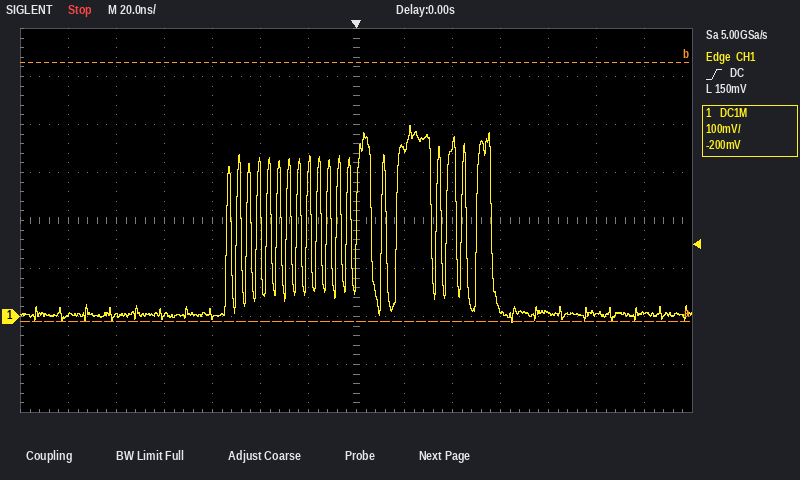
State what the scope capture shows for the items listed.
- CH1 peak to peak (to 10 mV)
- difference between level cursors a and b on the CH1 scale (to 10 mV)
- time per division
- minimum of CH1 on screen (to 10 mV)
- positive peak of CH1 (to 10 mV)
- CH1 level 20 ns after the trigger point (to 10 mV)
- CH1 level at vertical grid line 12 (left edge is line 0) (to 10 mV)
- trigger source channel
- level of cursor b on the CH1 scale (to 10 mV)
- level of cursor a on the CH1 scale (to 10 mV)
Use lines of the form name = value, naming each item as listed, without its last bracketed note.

CH1 peak to peak = 410 mV
difference between level cursors a and b on the CH1 scale = 540 mV
time per division = 20 ns
minimum of CH1 on screen = -10 mV
positive peak of CH1 = 400 mV
CH1 level 20 ns after the trigger point = 350 mV
CH1 level at vertical grid line 12 (left edge is line 0) = 0 mV
trigger source channel = CH1
level of cursor b on the CH1 scale = 530 mV
level of cursor a on the CH1 scale = -10 mV
